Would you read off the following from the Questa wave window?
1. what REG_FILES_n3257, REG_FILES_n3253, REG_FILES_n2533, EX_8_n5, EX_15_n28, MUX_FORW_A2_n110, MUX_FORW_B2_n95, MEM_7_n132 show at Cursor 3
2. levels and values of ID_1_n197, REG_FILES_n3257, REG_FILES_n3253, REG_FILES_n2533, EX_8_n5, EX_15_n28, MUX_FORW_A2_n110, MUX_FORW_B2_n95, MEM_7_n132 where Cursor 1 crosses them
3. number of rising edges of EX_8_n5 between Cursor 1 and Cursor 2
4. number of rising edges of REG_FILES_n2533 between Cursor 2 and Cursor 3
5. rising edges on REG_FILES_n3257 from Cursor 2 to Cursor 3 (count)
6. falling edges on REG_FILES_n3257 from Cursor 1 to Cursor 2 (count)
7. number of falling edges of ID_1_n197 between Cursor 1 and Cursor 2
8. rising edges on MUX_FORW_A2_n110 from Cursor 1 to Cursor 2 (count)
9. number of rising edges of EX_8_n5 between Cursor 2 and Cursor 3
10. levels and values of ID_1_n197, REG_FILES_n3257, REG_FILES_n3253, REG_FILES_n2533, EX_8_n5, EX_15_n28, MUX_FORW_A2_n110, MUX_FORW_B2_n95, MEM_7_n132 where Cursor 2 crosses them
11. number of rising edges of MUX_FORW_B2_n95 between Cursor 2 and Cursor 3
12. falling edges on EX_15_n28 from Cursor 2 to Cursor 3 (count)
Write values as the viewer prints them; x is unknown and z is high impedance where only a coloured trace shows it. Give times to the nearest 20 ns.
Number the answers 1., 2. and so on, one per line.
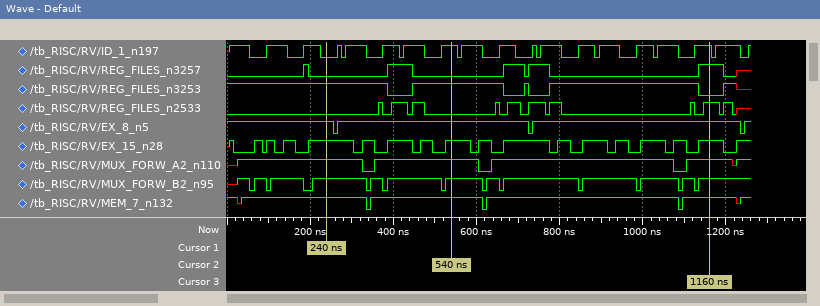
1. REG_FILES_n3257=1, REG_FILES_n3253=0, REG_FILES_n2533=1, EX_8_n5=1, EX_15_n28=1, MUX_FORW_A2_n110=1, MUX_FORW_B2_n95=1, MEM_7_n132=1
2. ID_1_n197=0, REG_FILES_n3257=0, REG_FILES_n3253=1, REG_FILES_n2533=0, EX_8_n5=1, EX_15_n28=1, MUX_FORW_A2_n110=1, MUX_FORW_B2_n95=1, MEM_7_n132=1
3. 1
4. 6
5. 3
6. 1
7. 4
8. 1
9. 1
10. ID_1_n197=1, REG_FILES_n3257=0, REG_FILES_n3253=1, REG_FILES_n2533=0, EX_8_n5=1, EX_15_n28=1, MUX_FORW_A2_n110=1, MUX_FORW_B2_n95=1, MEM_7_n132=1
11. 6
12. 8
